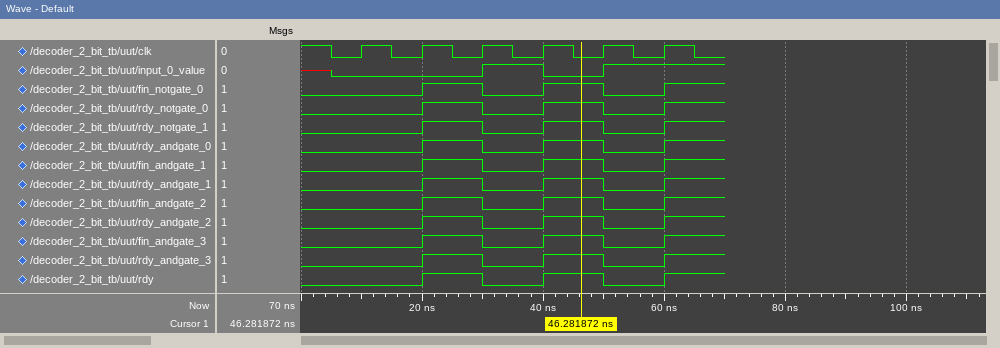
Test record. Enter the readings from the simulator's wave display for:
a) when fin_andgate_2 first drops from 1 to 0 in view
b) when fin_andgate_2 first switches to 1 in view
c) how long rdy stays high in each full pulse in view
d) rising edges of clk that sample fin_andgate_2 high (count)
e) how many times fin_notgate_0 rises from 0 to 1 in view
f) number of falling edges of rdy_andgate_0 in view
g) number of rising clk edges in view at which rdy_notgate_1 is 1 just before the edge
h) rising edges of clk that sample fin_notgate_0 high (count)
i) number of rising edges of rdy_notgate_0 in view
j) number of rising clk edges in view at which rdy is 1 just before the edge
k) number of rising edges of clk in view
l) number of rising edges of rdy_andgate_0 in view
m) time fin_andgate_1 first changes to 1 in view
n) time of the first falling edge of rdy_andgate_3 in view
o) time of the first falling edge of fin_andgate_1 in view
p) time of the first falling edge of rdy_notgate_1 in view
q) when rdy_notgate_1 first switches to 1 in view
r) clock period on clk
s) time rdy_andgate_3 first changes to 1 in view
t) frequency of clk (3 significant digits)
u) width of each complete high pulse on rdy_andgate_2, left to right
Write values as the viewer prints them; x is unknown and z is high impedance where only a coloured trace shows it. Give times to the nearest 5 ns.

30 ns
20 ns
10 ns, 10 ns
2
3
2
2
2
3
2
6
3
20 ns
30 ns
30 ns
30 ns
20 ns
10 ns
20 ns
100 MHz
10 ns, 10 ns
